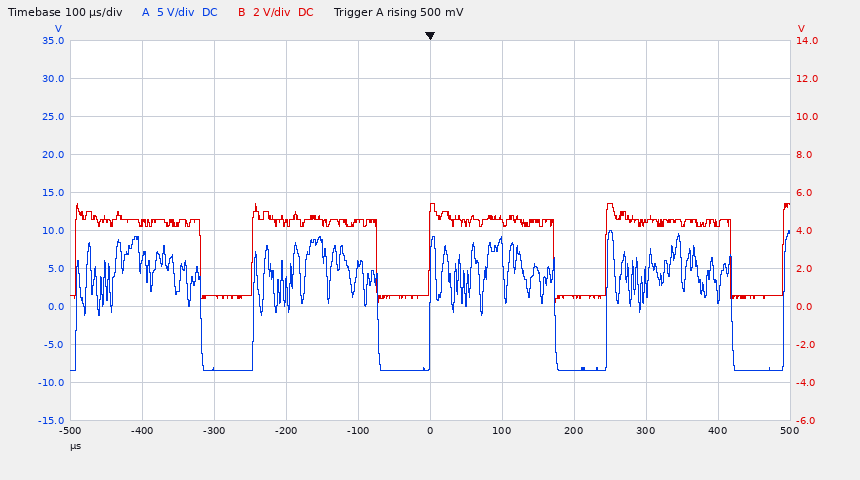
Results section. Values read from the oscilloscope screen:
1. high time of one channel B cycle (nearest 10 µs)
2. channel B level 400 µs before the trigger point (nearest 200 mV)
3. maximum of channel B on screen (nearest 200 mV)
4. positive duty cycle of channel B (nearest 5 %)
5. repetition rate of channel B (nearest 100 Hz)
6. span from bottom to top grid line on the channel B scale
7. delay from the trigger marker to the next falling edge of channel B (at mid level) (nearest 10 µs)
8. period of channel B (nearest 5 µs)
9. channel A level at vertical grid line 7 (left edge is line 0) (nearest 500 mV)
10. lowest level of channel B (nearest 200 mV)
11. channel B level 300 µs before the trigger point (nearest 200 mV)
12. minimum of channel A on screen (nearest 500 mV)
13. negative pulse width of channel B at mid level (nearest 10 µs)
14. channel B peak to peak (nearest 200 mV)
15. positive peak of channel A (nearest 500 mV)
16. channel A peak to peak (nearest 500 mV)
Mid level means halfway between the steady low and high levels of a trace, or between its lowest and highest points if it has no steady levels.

170 µs
4.4 V
5.4 V
70 %
4.1 kHz
20 V
170 µs
245 µs
-8.5 V
200 mV
600 mV
-8.5 V
70 µs
5.2 V
10.0 V
18.5 V
